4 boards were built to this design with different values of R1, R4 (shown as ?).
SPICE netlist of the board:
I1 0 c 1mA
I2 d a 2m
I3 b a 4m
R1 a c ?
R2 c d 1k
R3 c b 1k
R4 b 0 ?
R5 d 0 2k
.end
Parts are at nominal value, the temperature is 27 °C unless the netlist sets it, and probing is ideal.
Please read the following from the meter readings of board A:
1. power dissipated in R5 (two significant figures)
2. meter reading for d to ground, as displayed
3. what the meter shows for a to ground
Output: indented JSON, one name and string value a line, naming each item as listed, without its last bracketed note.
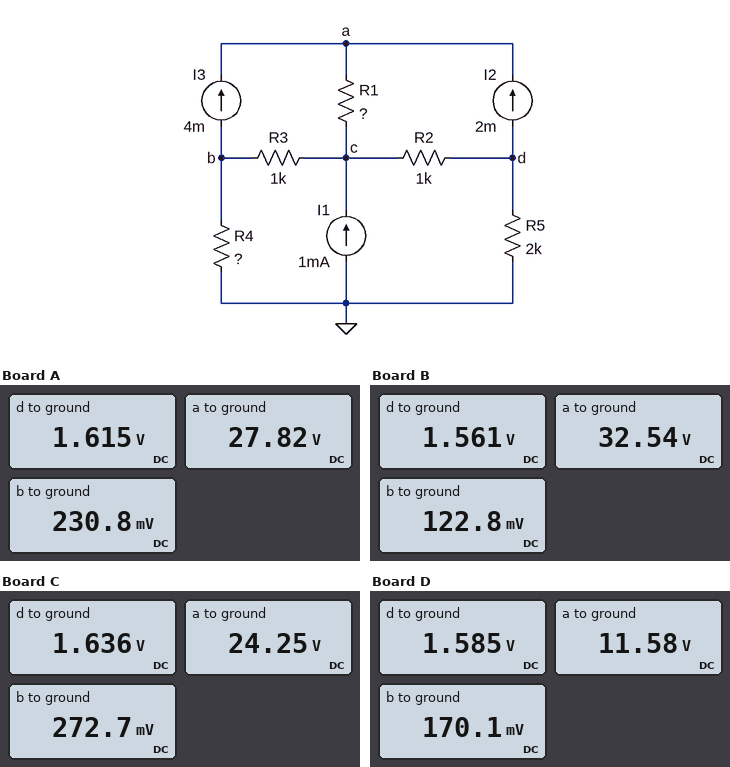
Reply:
{
  "power dissipated in R5": "1.3 mW",
  "meter reading for d to ground, as displayed": "1.615 V",
  "what the meter shows for a to ground": "27.82 V"
}
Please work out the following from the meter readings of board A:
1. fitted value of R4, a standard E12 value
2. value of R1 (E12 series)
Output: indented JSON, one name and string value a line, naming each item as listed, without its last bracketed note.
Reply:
{
  "fitted value of R4, a standard E12 value": "1.2 kΩ",
  "value of R1": "3.9 kΩ"
}
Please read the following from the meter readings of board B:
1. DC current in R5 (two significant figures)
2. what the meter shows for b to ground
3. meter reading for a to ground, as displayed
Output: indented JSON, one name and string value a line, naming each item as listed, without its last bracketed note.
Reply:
{
  "DC current in R5": "780 µA",
  "what the meter shows for b to ground": "122.8 mV",
  "meter reading for a to ground, as displayed": "32.54 V"
}
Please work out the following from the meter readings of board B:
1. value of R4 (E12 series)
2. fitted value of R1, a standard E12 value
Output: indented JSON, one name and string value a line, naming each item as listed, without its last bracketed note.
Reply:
{
  "value of R4": "560 Ω",
  "fitted value of R1, a standard E12 value": "4.7 kΩ"
}
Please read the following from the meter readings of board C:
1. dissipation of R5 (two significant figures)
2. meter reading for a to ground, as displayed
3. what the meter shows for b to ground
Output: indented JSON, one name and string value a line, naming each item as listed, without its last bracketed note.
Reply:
{
  "dissipation of R5": "1.3 mW",
  "meter reading for a to ground, as displayed": "24.25 V",
  "what the meter shows for b to ground": "272.7 mV"
}
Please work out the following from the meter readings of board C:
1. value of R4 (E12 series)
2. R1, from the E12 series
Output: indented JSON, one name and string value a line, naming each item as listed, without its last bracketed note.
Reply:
{
  "value of R4": "1.5 kΩ",
  "R1, from the E12 series": "3.3 kΩ"
}
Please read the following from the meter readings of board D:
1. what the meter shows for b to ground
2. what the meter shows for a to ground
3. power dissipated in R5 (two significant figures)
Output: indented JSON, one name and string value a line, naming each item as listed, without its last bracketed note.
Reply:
{
  "what the meter shows for b to ground": "170.1 mV",
  "what the meter shows for a to ground": "11.58 V",
  "power dissipated in R5": "1.3 mW"
}
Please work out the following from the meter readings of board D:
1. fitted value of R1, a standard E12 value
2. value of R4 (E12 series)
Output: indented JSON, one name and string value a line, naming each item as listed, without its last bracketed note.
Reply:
{
  "fitted value of R1, a standard E12 value": "1.2 kΩ",
  "value of R4": "820 Ω"
}
